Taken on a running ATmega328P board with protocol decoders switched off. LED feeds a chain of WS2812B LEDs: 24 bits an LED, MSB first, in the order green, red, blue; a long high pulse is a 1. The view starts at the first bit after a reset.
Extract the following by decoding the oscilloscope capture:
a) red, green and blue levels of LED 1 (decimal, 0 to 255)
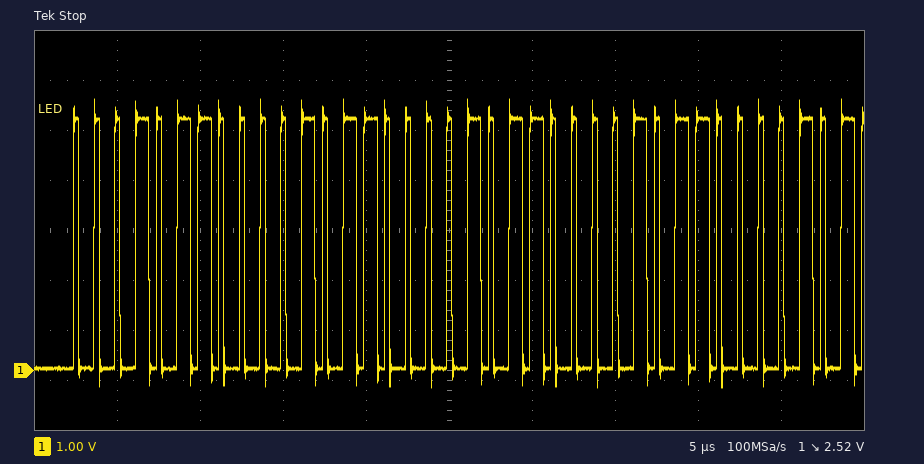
22, 22, 22
